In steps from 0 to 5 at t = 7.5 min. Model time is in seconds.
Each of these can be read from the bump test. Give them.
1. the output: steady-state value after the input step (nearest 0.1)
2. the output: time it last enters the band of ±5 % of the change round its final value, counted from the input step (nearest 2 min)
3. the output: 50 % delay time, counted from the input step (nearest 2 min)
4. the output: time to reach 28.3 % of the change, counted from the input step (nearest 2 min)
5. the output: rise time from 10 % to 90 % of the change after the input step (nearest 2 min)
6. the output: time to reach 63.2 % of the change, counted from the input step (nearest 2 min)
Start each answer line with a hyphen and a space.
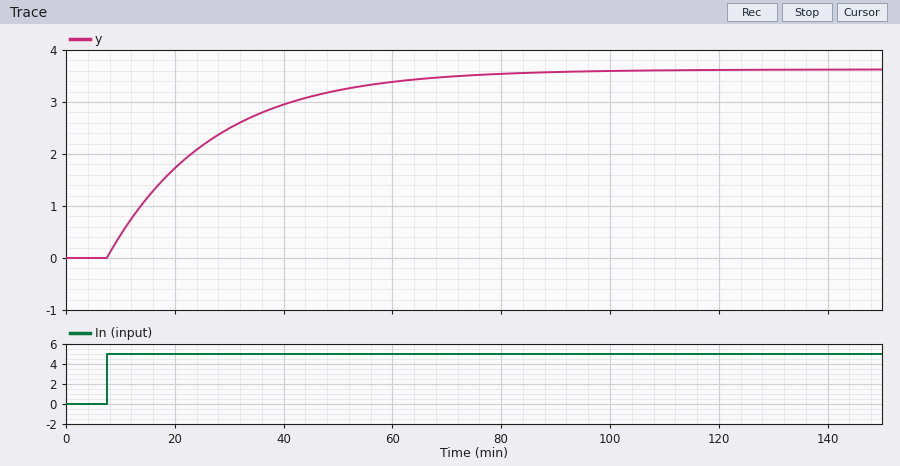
- 3.6
- 58 min
- 14 min
- 6 min
- 42 min
- 20 min
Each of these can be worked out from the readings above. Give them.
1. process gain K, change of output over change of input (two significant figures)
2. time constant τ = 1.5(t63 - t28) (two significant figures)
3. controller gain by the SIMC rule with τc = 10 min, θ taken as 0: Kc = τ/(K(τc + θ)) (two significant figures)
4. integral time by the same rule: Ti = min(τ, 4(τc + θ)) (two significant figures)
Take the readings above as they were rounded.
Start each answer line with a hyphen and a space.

- 0.72
- 21 min
- 2.9
- 21 min
